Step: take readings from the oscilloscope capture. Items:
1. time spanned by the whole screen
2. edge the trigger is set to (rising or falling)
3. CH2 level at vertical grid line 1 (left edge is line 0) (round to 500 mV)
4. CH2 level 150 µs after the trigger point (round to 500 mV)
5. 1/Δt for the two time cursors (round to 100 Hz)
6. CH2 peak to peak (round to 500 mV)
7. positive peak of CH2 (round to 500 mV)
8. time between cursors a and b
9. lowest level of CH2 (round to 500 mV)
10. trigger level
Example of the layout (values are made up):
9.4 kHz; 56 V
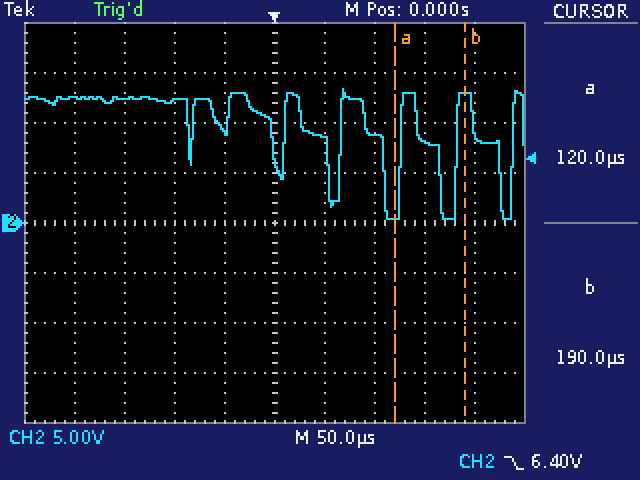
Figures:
500 µs; falling; 12.5 V; 8.0 V; 14.3 kHz; 13.0 V; 13.5 V; 70 µs; 500 mV; 6.40 V
